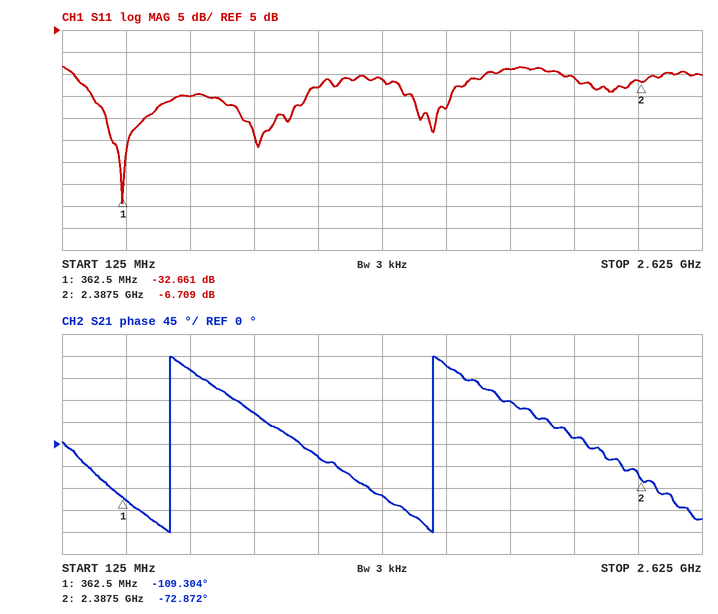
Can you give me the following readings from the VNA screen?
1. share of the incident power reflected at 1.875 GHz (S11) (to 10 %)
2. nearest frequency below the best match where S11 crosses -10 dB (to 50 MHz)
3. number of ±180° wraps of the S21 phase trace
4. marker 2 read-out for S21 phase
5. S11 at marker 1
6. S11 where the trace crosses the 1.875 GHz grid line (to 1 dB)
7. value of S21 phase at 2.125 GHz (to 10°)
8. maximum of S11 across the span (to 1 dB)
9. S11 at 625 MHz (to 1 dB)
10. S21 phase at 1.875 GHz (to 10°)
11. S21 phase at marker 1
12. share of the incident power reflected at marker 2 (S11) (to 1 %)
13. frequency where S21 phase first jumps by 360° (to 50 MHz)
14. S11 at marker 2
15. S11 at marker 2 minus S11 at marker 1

40 %
250 MHz
2
-72.872°
-32.661 dB
-4 dB
10°
-3 dB
-10 dB
90°
-109.304°
21 %
550 MHz
-6.709 dB
25.952 dB
